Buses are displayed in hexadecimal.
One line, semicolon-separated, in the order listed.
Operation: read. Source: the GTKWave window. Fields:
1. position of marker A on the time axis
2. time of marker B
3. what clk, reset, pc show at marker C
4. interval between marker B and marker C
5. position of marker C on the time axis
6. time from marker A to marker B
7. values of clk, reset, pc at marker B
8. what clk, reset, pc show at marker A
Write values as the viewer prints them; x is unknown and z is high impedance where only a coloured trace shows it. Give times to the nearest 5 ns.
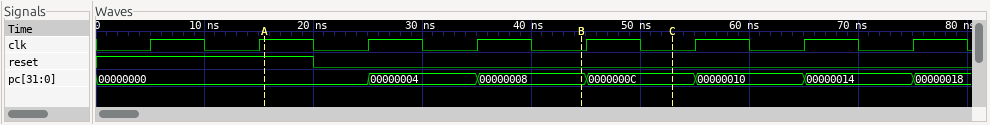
15 ns; 45 ns; clk=0, reset=0, pc=0000000C; 10 ns; 55 ns; 30 ns; clk=0, reset=0, pc=00000008; clk=1, reset=1, pc=00000000
